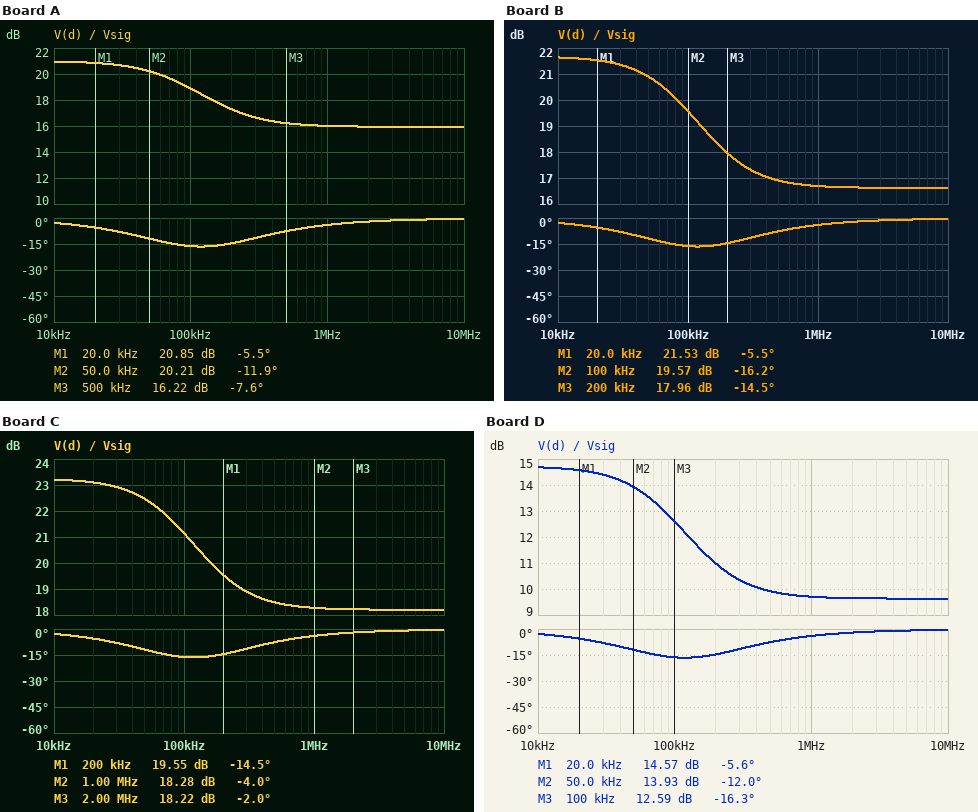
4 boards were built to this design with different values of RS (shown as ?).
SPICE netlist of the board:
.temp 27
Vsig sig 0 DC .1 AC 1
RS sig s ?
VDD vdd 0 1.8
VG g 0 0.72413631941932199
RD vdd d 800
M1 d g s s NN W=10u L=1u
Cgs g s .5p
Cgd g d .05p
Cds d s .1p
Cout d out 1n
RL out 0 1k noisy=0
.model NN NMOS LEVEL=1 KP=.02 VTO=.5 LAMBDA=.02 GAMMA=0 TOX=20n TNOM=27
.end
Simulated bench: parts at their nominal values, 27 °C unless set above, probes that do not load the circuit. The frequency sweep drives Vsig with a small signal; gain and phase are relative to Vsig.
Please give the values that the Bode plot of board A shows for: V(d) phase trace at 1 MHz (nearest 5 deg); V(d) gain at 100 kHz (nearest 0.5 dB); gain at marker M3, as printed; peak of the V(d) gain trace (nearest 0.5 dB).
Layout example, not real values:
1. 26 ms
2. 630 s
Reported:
1. -5 deg
2. 19.0 dB
3. 16.22 dB
4. 21.0 dB
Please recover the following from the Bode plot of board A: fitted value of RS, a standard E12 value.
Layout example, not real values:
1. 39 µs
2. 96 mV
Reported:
1. 22 Ω
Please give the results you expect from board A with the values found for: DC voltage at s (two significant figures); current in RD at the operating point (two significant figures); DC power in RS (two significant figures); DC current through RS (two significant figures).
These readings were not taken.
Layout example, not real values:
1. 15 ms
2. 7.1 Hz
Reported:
1. 120 mV
2. 1.0 mA
3. 24 µW
4. 1.0 mA
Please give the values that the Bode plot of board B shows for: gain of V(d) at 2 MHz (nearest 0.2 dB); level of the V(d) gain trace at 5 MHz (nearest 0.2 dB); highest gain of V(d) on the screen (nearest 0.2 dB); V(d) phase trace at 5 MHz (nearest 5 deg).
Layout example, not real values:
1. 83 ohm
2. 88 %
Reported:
1. 16.6 dB
2. 16.6 dB
3. 21.6 dB
4. 0 deg
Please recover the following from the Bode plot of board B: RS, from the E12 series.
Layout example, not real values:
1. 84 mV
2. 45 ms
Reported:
1. 18 Ω
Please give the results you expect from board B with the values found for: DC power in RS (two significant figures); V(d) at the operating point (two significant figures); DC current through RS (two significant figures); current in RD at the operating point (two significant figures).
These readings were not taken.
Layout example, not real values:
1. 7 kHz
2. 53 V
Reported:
1. 22 µW
2. 920 mV
3. 1.1 mA
4. 1.1 mA
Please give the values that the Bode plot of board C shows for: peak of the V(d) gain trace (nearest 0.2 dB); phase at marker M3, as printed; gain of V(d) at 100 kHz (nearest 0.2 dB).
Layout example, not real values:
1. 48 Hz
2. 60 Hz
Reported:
1. 23.2 dB
2. -2.0 deg
3. 21.2 dB
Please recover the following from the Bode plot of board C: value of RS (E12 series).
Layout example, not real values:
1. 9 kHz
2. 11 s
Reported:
1. 10 Ω
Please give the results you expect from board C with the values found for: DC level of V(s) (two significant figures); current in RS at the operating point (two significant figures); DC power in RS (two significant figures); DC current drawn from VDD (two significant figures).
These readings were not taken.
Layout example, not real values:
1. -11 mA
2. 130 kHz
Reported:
1. 110 mV
2. 1.3 mA
3. 16 µW
4. 1.3 mA
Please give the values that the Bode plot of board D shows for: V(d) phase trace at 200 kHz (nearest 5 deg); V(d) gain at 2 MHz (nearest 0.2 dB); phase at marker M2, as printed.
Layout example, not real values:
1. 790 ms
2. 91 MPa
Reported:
1. -15 deg
2. 9.6 dB
3. -12.0 deg
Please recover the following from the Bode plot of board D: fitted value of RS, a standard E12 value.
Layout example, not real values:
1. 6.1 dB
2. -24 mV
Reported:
1. 82 Ω
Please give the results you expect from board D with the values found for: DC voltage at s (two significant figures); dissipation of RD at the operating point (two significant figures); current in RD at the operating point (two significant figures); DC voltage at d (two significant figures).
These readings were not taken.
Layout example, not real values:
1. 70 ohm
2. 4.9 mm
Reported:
1. 150 mV
2. 280 µW
3. 590 µA
4. 1.3 V
